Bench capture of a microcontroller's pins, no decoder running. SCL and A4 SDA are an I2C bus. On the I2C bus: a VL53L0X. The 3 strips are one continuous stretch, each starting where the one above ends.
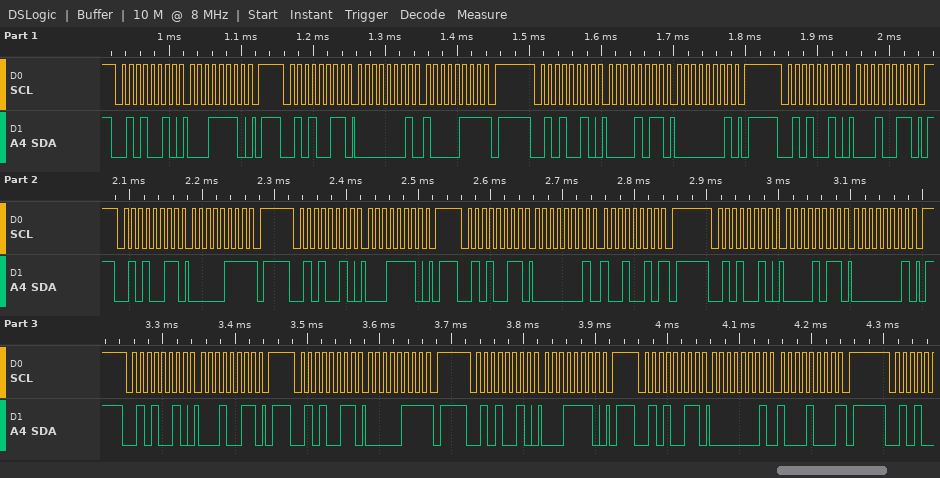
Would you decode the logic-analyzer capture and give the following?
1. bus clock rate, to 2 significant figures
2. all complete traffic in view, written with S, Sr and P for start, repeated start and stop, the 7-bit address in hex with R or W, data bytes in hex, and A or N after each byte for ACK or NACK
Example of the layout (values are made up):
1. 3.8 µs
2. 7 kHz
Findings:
1. 100 kHz
2. S 29W A 1E A P S 29R A 01 A 87 N P S 29W A 0B A 01 A P S 29W A 13 A P S 29R A 07 N P S 29W A 1E A P S 29R A 01 A 92 N P S 29W A 0B A 01 A P S 29W A 13 A P S 29R A 07 N P S 29W A 1E A P S 29R A 01 A 88 N P
